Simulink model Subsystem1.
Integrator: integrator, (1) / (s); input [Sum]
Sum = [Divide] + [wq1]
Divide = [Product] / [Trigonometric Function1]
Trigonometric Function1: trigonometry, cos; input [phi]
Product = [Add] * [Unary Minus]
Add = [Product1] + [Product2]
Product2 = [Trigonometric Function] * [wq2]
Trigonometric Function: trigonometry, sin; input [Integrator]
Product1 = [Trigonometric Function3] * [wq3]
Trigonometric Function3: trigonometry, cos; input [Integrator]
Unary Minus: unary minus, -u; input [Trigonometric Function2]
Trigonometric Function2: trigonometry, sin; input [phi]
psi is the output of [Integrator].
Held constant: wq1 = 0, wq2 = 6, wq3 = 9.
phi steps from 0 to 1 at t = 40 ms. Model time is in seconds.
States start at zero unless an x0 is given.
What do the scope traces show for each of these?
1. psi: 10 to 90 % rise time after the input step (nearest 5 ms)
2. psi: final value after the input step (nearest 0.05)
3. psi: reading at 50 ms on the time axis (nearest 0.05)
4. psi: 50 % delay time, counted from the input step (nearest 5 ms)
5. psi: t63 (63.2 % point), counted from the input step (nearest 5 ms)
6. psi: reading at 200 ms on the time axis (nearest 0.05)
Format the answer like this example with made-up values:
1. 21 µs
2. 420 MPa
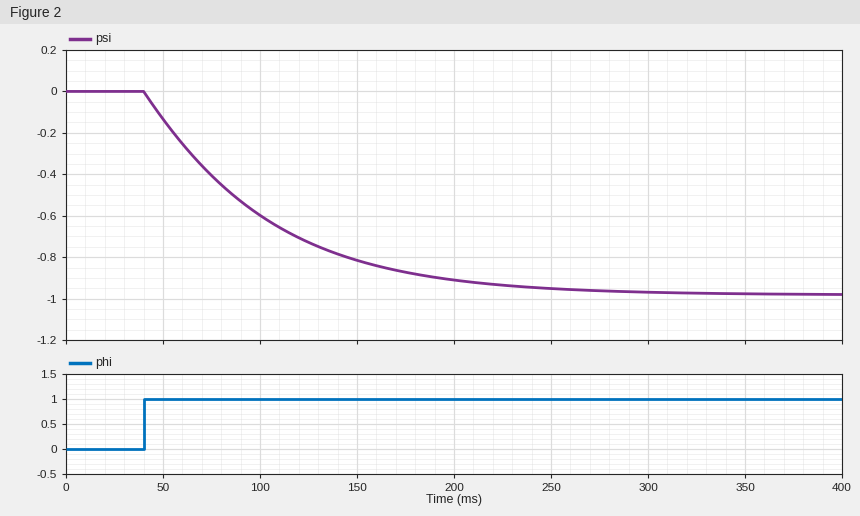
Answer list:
1. 135 ms
2. -1.00
3. -0.15
4. 45 ms
5. 65 ms
6. -0.90
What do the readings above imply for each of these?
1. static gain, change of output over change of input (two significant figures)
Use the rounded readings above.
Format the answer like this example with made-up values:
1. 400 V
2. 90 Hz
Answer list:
1. -1.0
